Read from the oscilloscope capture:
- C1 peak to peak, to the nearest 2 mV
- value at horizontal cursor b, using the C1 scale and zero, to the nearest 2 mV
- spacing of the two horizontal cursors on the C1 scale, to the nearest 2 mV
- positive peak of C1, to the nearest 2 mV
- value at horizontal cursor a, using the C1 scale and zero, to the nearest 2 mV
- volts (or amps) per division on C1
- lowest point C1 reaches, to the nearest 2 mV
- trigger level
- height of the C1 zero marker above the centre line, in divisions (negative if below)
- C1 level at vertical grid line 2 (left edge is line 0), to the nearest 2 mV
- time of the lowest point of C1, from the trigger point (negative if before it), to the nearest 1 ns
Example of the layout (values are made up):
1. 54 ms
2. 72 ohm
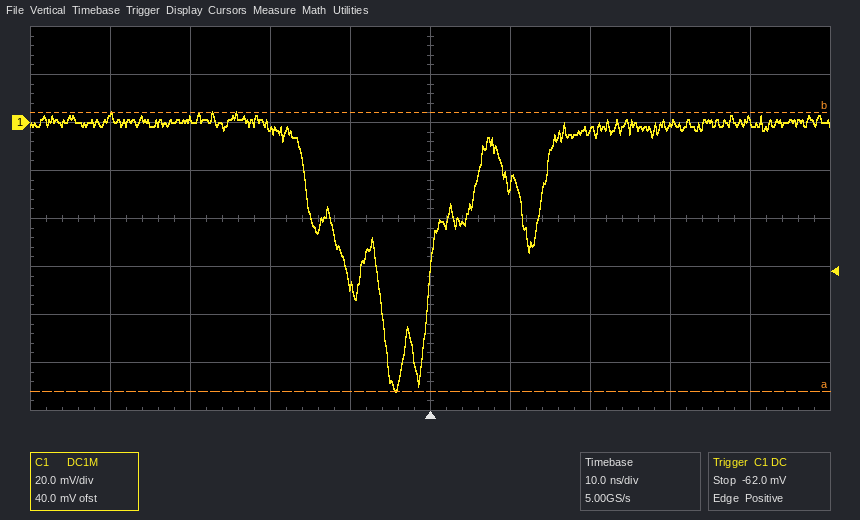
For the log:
1. 116 mV
2. 4 mV
3. 116 mV
4. 4 mV
5. -112 mV
6. 20 mV
7. -112 mV
8. -62.0 mV
9. +2.0 div
10. 2 mV
11. -4 ns
